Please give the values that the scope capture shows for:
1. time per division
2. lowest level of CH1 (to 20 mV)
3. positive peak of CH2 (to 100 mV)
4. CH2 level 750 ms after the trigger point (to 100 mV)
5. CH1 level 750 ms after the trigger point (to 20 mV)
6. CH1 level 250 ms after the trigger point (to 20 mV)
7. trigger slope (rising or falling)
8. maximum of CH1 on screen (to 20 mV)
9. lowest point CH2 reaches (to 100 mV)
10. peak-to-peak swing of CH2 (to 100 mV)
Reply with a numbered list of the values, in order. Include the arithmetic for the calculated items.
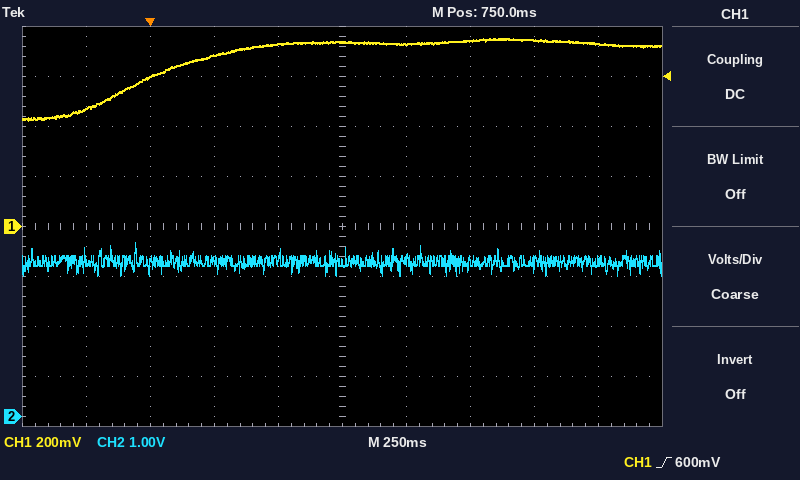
1. 250 ms
2. 420 mV
3. 3.5 V
4. 3.1 V
5. 740 mV
6. 680 mV
7. rising
8. 760 mV
9. 2.8 V
10. 3.5 V − (2.8 V) = 700 mV
